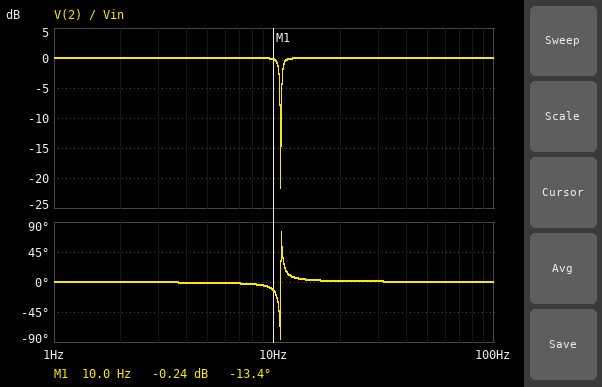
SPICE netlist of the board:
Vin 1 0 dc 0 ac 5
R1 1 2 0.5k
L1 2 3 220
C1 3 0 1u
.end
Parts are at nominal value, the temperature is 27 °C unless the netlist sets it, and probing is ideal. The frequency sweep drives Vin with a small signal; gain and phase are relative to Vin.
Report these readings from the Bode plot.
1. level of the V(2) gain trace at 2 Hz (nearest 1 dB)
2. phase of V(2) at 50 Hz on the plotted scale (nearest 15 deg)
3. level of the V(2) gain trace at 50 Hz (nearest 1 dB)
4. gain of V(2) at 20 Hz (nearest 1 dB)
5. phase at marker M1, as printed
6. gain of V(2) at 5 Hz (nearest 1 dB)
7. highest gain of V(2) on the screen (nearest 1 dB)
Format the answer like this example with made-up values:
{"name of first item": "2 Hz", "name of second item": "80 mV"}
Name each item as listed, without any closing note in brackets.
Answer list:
{"level of the V(2) gain trace at 2 Hz": "0 dB", "phase of V(2) at 50 Hz on the plotted scale": "0 deg", "level of the V(2) gain trace at 50 Hz": "0 dB", "gain of V(2) at 20 Hz": "0 dB", "phase at marker M1, as printed": "-13.4 deg", "gain of V(2) at 5 Hz": "0 dB", "highest gain of V(2) on the screen": "0 dB"}
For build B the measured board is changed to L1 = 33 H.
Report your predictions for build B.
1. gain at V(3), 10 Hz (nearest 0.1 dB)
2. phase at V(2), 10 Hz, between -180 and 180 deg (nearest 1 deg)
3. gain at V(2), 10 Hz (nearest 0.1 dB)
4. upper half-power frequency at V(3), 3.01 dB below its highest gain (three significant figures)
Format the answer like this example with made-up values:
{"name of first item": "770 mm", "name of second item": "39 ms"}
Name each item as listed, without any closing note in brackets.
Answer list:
{"gain at V(3), 10 Hz": "1.2 dB", "phase at V(2), 10 Hz, between -180 and 180 deg": "-2 deg", "gain at V(2), 10 Hz": "0 dB", "upper half-power frequency at V(3), 3.01 dB below its highest gain": "28.8 Hz"}
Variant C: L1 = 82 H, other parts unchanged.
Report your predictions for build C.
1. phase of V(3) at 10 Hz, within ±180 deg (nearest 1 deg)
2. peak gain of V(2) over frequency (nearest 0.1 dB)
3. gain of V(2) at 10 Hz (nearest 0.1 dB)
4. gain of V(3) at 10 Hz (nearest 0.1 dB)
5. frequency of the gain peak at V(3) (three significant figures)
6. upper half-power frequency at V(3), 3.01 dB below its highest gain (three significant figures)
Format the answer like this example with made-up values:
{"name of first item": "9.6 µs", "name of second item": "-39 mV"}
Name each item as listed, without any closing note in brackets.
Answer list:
{"phase of V(3) at 10 Hz, within ±180 deg": "-3 deg", "peak gain of V(2) over frequency": "0 dB", "gain of V(2) at 10 Hz": "0 dB", "gain of V(3) at 10 Hz": "3.4 dB", "frequency of the gain peak at V(3)": "17.6 Hz", "upper half-power frequency at V(3), 3.01 dB below its highest gain": "18.0 Hz"}
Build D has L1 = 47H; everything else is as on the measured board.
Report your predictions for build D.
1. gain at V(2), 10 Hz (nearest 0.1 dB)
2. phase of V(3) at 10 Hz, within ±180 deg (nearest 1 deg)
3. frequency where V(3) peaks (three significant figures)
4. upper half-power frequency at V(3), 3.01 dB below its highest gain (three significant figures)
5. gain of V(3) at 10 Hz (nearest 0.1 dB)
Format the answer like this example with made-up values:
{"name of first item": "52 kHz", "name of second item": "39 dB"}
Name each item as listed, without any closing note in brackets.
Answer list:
{"gain at V(2), 10 Hz": "0 dB", "phase of V(3) at 10 Hz, within ±180 deg": "-2 deg", "frequency where V(3) peaks": "23.2 Hz", "upper half-power frequency at V(3), 3.01 dB below its highest gain": "24.0 Hz", "gain of V(3) at 10 Hz": "1.8 dB"}
